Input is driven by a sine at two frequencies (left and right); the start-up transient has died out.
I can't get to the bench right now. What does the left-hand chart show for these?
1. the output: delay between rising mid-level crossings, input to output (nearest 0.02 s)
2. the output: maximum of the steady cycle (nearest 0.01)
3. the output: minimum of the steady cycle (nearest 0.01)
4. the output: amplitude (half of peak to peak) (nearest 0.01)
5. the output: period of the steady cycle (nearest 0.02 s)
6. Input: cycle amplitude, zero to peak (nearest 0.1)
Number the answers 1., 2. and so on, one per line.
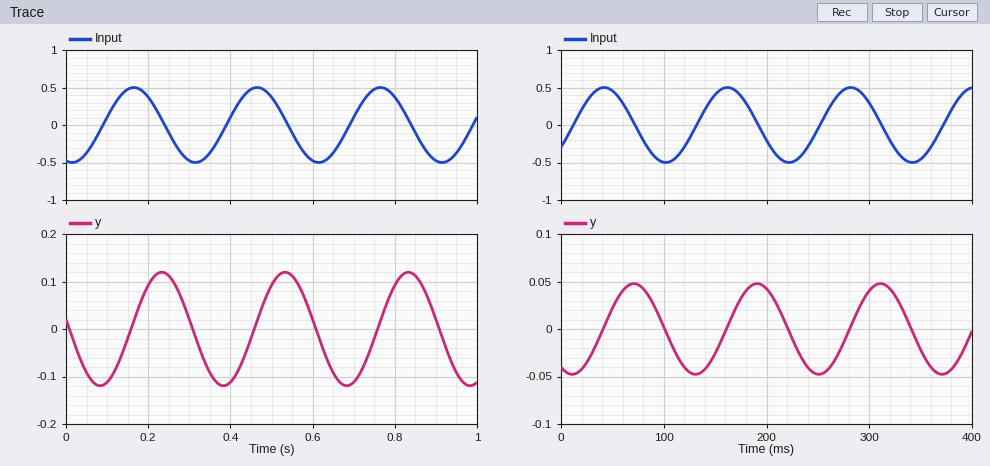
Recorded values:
1. 0.06 s
2. 0.12
3. -0.12
4. 0.12
5. 0.30 s
6. 0.5
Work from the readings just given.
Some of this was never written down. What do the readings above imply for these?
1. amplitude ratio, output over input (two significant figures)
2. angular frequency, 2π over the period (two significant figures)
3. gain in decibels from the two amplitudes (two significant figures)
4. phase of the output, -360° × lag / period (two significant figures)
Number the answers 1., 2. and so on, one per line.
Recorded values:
1. 0.24
2. 21 rad/s
3. -12 dB
4. -72°
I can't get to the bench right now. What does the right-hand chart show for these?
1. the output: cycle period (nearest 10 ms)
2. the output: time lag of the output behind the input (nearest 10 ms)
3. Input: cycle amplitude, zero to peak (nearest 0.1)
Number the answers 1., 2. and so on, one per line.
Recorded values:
1. 120 ms
2. 30 ms
3. 0.5
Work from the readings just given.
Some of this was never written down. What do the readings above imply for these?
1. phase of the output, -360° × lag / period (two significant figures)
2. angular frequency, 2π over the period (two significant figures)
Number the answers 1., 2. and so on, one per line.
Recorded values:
1. -90°
2. 0.052 rad/ms
